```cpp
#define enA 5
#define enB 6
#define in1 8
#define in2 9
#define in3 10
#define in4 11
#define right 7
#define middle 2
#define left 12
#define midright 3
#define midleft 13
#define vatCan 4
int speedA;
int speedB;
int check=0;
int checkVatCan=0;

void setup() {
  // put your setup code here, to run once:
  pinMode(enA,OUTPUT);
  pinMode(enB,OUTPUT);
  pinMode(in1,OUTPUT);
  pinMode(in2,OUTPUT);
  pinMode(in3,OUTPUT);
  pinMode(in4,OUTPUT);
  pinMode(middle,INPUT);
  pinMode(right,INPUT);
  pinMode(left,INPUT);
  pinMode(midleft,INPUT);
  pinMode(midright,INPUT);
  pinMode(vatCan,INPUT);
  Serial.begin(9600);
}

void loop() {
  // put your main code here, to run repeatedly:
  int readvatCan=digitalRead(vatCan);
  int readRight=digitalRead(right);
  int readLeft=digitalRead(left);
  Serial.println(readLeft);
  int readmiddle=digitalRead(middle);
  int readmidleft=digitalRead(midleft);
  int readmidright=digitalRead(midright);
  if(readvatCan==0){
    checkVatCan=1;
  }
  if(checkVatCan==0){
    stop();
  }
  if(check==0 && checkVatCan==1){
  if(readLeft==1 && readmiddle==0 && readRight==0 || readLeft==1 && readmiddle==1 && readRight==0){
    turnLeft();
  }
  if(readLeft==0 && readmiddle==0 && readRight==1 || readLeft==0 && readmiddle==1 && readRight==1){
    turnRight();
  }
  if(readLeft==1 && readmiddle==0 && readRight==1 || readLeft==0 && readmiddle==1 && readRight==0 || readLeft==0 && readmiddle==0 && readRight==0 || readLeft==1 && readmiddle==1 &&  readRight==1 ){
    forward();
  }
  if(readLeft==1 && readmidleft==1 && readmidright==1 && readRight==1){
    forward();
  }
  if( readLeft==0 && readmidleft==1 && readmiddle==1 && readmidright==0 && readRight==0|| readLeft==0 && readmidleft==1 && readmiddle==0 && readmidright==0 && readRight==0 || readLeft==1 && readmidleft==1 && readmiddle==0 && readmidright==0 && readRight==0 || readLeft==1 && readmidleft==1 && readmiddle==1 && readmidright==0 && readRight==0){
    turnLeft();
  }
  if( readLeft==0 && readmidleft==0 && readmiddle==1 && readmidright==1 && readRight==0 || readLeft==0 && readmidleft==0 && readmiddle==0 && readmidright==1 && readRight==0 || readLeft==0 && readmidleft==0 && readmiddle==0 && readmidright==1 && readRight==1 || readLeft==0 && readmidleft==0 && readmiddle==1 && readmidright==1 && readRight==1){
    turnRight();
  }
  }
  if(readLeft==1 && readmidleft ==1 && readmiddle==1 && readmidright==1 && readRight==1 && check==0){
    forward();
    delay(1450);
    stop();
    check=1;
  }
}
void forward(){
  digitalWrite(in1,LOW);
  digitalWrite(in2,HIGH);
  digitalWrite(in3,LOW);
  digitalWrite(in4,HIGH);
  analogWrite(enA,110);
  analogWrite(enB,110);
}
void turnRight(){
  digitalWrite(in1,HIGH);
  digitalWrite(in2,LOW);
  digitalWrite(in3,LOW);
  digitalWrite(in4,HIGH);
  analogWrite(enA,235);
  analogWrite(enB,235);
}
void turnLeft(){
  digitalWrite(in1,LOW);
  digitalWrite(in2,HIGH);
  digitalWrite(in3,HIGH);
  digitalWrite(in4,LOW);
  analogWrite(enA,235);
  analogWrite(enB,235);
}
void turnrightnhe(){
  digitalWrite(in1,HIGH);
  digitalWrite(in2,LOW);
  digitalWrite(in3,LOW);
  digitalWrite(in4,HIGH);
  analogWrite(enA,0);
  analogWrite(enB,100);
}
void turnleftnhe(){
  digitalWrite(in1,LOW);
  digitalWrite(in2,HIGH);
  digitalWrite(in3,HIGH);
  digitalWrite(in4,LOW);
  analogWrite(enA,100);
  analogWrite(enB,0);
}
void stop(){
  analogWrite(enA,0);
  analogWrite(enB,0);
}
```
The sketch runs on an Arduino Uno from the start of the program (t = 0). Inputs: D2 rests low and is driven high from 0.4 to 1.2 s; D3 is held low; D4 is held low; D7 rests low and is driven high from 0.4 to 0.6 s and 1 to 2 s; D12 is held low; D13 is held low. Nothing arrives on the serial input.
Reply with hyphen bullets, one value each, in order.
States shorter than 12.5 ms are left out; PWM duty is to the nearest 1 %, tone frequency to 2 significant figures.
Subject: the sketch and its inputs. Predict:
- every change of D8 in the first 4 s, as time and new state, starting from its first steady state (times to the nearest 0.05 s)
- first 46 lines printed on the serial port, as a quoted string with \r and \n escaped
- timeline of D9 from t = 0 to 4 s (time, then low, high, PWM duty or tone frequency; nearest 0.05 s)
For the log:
- 0 s low; 0.4 s high; 0.6 s low; 1 s high; 2 s low
- "0\r\n0\r\n0\r\n0\r\n0\r\n0\r\n0\r\n0\r\n0\r\n0\r\n0\r\n0\r\n0\r\n0\r\n0\r\n0\r\n0\r\n0\r\n0\r\n0\r\n0\r\n0\r\n0\r\n0\r\n0\r\n0\r\n0\r\n0\r\n0\r\n0\r\n0\r\n0\r\n0\r\n0\r\n0\r\n0\r\n0\r\n0\r\n0\r\n0\r\n0\r\n0\r\n0\r\n0\r\n0\r\n0\r\n"
- 0 s high; 0.4 s low; 0.6 s high; 1 s low; 2 s high
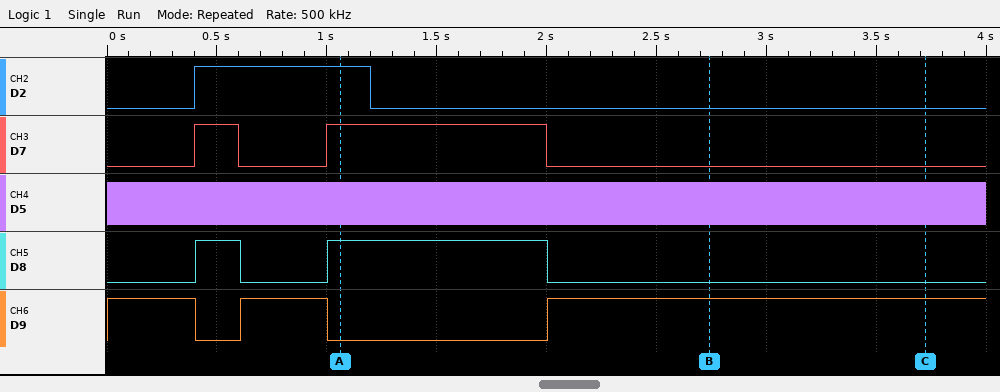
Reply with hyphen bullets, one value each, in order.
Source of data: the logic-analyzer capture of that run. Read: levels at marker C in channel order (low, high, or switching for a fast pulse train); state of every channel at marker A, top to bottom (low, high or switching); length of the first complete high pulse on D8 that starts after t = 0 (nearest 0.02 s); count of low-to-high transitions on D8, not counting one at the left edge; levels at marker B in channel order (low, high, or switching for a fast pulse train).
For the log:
- D2 low, D7 low, D5 switching, D8 low, D9 high
- D2 high, D7 high, D5 switching, D8 high, D9 low
- 0.20 s
- 2
- D2 low, D7 low, D5 switching, D8 low, D9 high
